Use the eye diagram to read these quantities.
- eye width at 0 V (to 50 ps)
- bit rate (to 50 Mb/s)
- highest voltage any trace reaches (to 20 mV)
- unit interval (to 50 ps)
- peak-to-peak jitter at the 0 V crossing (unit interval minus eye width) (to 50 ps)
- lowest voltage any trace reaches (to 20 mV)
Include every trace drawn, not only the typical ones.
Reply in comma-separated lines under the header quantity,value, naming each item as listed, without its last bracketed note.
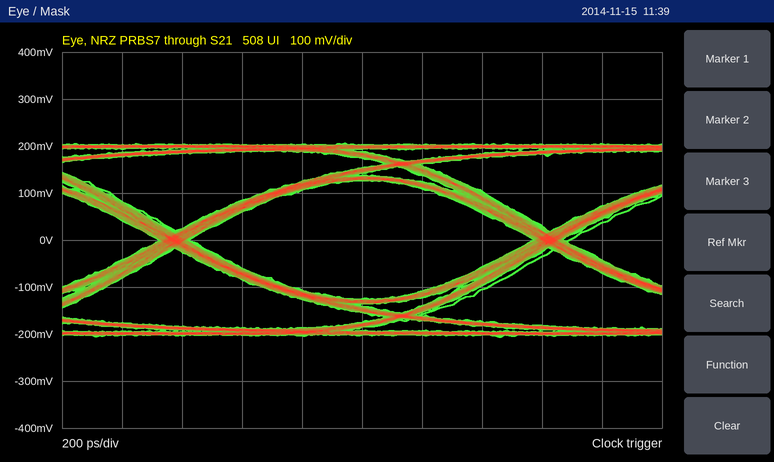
quantity,value
eye width at 0 V,1.15 ns
bit rate,800 Mb/s
highest voltage any trace reaches,200 mV
unit interval,1.25 ns
peak-to-peak jitter at the 0 V crossing (unit interval minus eye width),100 ps
lowest voltage any trace reaches,-200 mV
